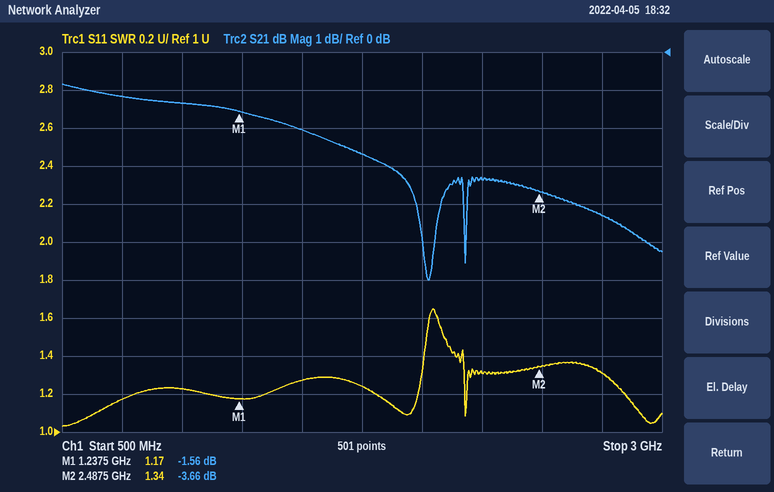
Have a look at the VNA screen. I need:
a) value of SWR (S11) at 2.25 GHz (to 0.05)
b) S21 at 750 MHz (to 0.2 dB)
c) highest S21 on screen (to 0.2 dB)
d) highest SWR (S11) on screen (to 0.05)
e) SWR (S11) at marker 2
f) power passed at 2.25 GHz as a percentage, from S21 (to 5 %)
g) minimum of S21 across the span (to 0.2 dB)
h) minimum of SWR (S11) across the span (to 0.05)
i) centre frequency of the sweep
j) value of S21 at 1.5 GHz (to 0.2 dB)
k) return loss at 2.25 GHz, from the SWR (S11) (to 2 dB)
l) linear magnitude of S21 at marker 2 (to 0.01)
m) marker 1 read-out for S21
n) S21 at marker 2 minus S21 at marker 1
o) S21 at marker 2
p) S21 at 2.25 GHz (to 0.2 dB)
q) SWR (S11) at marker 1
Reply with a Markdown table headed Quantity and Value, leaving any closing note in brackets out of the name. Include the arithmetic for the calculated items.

| Quantity | Value |
|---|---|
| value of SWR (S11) at 2.25 GHz | 1.30 |
| S21 at 750 MHz | -1.2 dB |
| highest S21 on screen | -0.8 dB |
| highest SWR (S11) on screen | 1.65 |
| SWR (S11) at marker 2 | 1.34 |
| power passed at 2.25 GHz as a percentage, from S21 | 10^(-3.4/10) ≈ 45.7 %, so 45 % to the nearest 5 % |
| minimum of S21 across the span | -6.0 dB |
| minimum of SWR (S11) across the span | 1.05 |
| centre frequency of the sweep | 1.75 GHz |
| value of S21 at 1.5 GHz | -2.0 dB |
| return loss at 2.25 GHz, from the SWR (S11) | −20 log10((1.3 − 1)/(1.3 + 1)) ≈ 18 dB |
| linear magnitude of S21 at marker 2 | 10^(-3.66/20) ≈ 0.66 |
| marker 1 read-out for S21 | -1.56 dB |
| S21 at marker 2 minus S21 at marker 1 | -3.66 − (-1.56) = -2.10 dB |
| S21 at marker 2 | -3.66 dB |
| S21 at 2.25 GHz | -3.4 dB |
| SWR (S11) at marker 1 | 1.17 |
